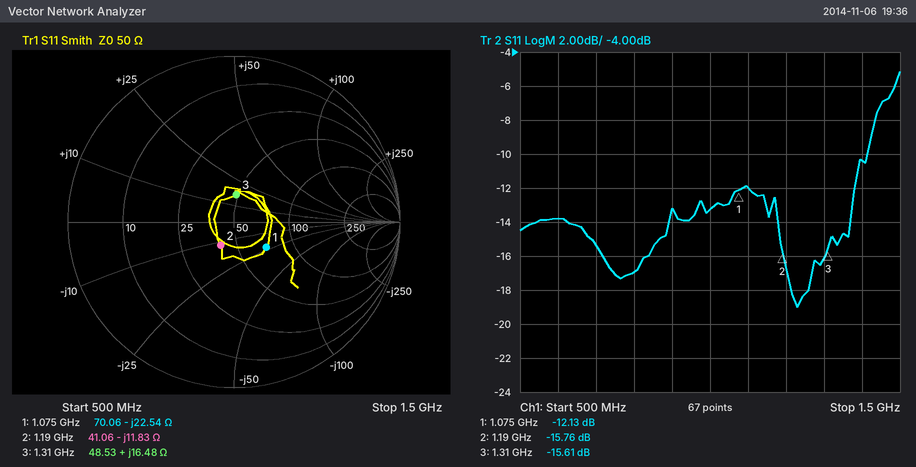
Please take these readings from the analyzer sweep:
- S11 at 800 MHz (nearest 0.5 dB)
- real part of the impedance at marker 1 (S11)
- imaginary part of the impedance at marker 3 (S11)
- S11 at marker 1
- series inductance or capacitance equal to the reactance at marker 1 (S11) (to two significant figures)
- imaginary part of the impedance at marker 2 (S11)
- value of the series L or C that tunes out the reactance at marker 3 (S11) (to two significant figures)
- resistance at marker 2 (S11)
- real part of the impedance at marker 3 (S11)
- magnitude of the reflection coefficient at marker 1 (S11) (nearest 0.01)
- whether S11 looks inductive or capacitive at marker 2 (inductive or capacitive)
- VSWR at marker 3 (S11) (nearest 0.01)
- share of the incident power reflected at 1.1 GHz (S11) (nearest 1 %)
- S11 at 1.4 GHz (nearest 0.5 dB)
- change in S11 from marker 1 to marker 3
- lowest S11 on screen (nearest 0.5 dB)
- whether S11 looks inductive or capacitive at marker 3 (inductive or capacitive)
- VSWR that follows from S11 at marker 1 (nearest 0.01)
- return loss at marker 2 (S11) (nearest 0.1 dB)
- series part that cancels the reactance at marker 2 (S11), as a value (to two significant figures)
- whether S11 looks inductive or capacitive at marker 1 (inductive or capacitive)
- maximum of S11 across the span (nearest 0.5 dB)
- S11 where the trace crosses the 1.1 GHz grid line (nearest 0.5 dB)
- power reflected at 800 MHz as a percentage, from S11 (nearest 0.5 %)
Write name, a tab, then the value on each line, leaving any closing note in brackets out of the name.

S11 at 800 MHz	-17.0 dB
real part of the impedance at marker 1	70.06 Ω
imaginary part of the impedance at marker 3	+16.48 Ω
S11 at marker 1	-12.13 dB
series inductance or capacitance equal to the reactance at marker 1 (S11)	6.6 pF
imaginary part of the impedance at marker 2	-11.83 Ω
value of the series L or C that tunes out the reactance at marker 3 (S11)	7.4 pF
resistance at marker 2	41.06 Ω
real part of the impedance at marker 3	48.53 Ω
magnitude of the reflection coefficient at marker 1 (S11)	0.25
whether S11 looks inductive or capacitive at marker 2	capacitive
VSWR at marker 3 (S11)	1.40
share of the incident power reflected at 1.1 GHz (S11)	6 %
S11 at 1.4 GHz	-10.5 dB
change in S11 from marker 1 to marker 3	-3.48 dB
lowest S11 on screen	-19.0 dB
whether S11 looks inductive or capacitive at marker 3	inductive
VSWR that follows from S11 at marker 1	1.66
return loss at marker 2 (S11)	15.8 dB
series part that cancels the reactance at marker 2 (S11), as a value	1.6 nH
whether S11 looks inductive or capacitive at marker 1	capacitive
maximum of S11 across the span	-5.0 dB
S11 where the trace crosses the 1.1 GHz grid line	-12.0 dB
power reflected at 800 MHz as a percentage, from S11	2.0 %
